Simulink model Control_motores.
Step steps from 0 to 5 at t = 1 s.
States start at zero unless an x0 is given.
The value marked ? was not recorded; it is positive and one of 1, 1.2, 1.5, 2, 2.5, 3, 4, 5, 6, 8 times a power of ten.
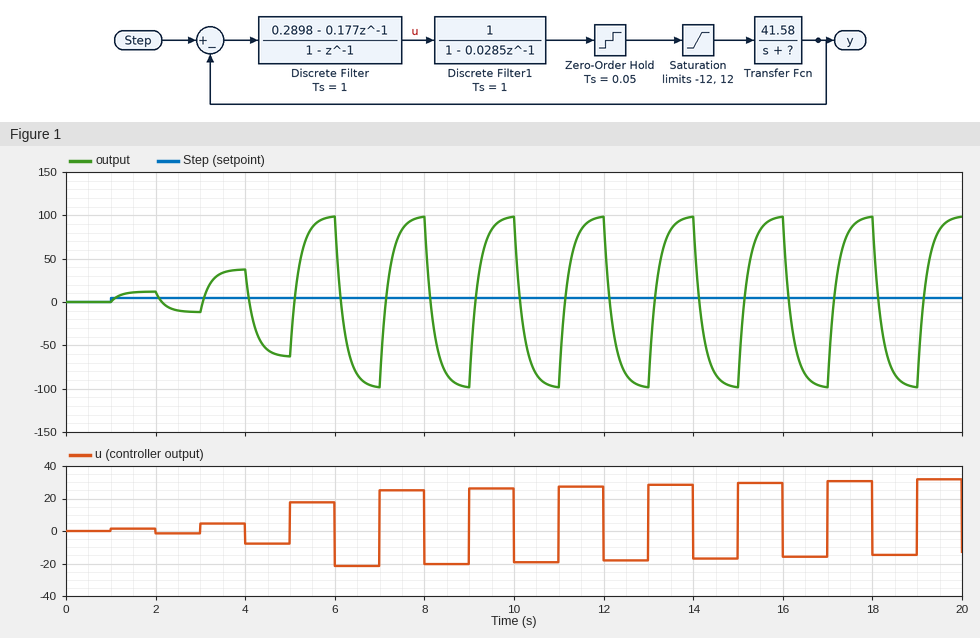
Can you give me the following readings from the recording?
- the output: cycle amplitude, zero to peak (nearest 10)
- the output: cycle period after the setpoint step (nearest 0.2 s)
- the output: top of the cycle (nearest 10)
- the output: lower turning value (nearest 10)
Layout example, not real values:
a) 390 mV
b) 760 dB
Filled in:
a) 100
b) 2.0 s
c) 100
d) -100
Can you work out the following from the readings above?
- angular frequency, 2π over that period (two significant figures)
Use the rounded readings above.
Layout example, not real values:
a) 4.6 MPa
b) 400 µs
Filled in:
a) 3.1 rad/s
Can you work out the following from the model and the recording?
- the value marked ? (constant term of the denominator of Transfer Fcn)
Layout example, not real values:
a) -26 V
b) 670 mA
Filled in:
a) 5
